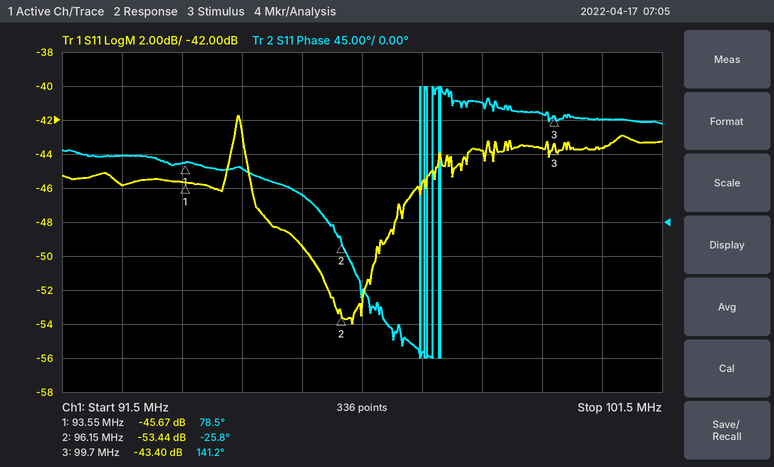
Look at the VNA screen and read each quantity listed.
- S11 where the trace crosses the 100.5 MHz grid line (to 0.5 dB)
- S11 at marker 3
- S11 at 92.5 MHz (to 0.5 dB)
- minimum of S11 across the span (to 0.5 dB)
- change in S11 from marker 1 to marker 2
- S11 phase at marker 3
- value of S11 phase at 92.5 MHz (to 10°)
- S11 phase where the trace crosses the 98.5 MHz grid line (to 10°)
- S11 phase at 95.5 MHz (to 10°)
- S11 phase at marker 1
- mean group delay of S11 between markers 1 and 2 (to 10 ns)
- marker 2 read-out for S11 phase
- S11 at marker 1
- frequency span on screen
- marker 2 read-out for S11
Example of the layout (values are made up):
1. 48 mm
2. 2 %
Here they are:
1. -43.5 dB
2. -43.40 dB
3. -46.0 dB
4. -54.0 dB
5. -7.77 dB
6. 141.2°
7. 90°
8. 160°
9. 40°
10. 78.5°
11. 110 ns
12. -25.8°
13. -45.67 dB
14. 10 MHz
15. -53.44 dB
